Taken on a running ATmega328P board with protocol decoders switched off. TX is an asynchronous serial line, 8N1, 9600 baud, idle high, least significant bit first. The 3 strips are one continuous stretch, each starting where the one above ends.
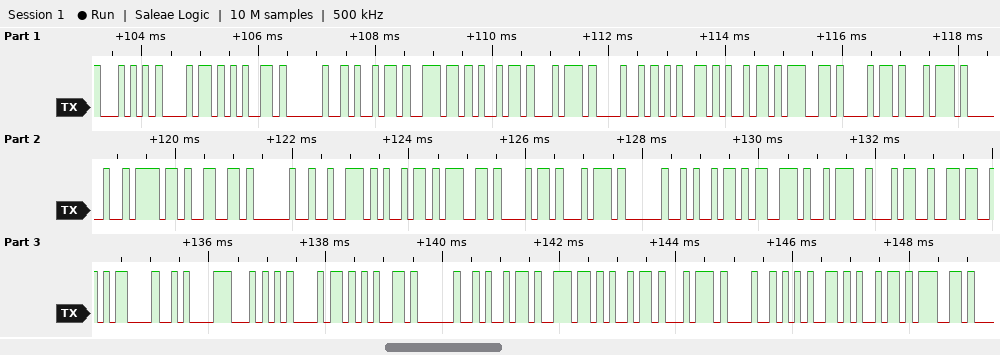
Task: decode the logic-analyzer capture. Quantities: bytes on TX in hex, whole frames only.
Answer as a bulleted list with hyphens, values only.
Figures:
- 54 68 65 20 69 6E 69 74 48 65 69 67 68 74 20 6F 66 20 72 69 67 68 74 20 69 73 3A 34 36 0D 0A 54 68 65 20 69 6E 69 74 48 65 69 67
